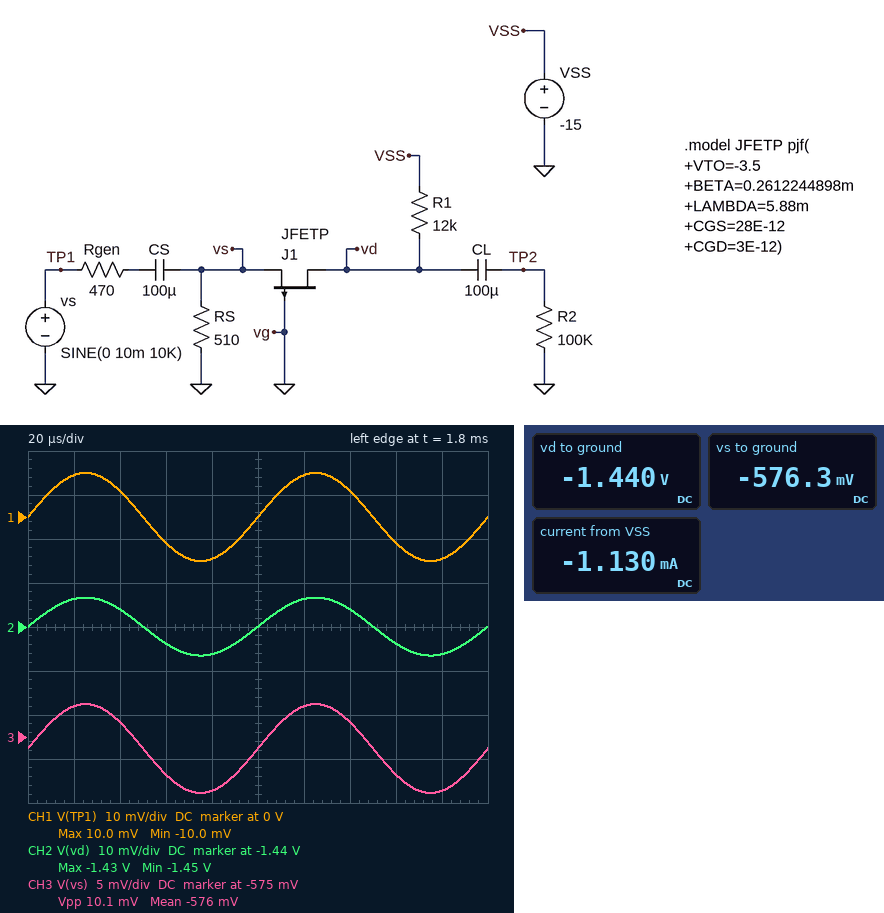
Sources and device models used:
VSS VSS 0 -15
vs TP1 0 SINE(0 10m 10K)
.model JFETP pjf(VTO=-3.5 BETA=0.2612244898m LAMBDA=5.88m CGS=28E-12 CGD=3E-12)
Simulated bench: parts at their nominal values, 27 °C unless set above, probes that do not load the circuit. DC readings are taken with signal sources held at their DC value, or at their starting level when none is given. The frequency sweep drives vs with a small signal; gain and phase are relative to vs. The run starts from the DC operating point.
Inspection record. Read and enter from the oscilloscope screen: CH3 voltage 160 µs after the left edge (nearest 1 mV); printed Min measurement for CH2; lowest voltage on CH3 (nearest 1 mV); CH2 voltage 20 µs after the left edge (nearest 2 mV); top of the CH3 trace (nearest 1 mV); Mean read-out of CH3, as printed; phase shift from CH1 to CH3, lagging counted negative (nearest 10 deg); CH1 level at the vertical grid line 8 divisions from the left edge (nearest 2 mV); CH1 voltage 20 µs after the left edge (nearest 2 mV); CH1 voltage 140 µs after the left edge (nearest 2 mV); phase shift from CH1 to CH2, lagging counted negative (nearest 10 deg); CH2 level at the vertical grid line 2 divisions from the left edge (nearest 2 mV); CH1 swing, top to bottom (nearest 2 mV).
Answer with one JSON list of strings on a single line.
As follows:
["-579 mV", "-1.45 V", "-581 mV", "-1.434 V", "-571 mV", "-576 mV", "0 deg", "-6 mV", "10 mV", "6 mV", "0 deg", "-1.436 V", "20 mV"]
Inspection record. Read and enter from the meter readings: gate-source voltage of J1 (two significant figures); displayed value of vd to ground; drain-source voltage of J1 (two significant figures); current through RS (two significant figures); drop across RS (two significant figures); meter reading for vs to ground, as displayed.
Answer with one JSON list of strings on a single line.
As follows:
["580 mV", "-1.440 V", "-860 mV", "1.1 mA", "580 mV", "-576.3 mV"]
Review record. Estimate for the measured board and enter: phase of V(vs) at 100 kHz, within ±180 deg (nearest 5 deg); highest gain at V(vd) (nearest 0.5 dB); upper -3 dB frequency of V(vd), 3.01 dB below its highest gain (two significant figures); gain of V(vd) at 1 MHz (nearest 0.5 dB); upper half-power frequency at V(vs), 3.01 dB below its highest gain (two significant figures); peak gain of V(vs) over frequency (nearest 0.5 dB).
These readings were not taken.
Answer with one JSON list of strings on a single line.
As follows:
["0 deg", "-3.5 dB", "25 MHz", "-3.5 dB", "27 MHz", "-6.0 dB"]
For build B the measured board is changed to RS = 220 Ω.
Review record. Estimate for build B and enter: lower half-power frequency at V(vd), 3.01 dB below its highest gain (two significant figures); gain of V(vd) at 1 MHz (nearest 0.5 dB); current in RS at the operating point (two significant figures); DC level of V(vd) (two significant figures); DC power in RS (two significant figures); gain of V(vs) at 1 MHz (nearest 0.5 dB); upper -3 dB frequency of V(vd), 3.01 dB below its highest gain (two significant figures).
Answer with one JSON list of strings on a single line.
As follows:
["2.3 Hz", "-8.5 dB", "1.2 mA", "-1.0 V", "300 µW", "-10.0 dB", "35 MHz"]
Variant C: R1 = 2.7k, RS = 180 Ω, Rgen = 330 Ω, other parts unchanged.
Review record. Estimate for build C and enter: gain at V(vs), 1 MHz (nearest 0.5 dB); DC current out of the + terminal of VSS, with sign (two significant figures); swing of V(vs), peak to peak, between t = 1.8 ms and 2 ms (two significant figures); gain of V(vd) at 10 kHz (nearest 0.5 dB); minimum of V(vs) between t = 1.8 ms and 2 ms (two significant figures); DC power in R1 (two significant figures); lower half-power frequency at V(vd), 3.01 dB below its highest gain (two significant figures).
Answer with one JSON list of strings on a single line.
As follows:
["-10.5 dB", "-2.5 mA", "5.9 mV", "2.0 dB", "-460 mV", "17 mW", "3.4 Hz"]
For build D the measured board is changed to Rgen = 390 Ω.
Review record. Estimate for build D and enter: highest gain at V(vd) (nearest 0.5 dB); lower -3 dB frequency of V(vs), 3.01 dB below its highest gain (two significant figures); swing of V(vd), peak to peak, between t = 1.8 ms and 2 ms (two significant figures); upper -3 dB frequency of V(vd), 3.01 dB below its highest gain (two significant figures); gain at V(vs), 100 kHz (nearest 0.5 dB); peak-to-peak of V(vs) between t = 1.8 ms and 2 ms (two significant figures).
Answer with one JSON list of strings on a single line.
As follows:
["-3.0 dB", "1.8 Hz", "14 mV", "27 MHz", "-5.0 dB", "11 mV"]
